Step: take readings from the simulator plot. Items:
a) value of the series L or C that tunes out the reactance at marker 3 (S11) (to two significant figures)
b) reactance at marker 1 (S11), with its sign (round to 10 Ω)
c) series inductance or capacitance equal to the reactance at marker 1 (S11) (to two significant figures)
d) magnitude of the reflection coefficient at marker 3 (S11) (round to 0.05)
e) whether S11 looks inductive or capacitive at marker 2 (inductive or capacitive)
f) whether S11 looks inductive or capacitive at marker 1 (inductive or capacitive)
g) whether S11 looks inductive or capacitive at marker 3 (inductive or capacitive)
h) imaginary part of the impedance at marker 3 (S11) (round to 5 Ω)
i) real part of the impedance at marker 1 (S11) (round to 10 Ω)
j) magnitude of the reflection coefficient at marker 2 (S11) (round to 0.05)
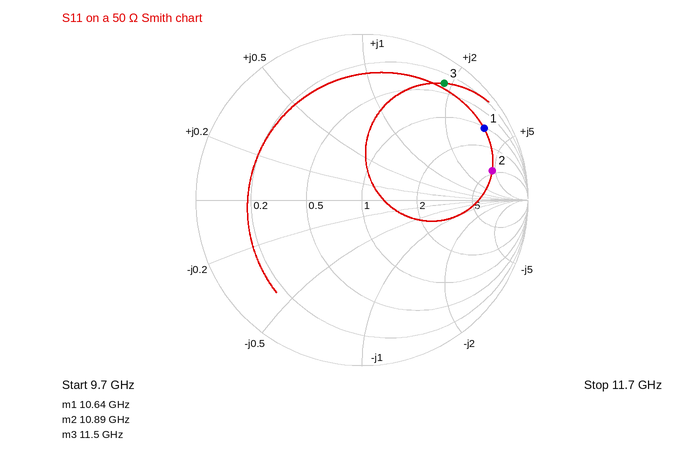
150 fF
+170 Ω
2.5 nH
0.85
inductive
inductive
inductive
+95 Ω
50 Ω
0.80
